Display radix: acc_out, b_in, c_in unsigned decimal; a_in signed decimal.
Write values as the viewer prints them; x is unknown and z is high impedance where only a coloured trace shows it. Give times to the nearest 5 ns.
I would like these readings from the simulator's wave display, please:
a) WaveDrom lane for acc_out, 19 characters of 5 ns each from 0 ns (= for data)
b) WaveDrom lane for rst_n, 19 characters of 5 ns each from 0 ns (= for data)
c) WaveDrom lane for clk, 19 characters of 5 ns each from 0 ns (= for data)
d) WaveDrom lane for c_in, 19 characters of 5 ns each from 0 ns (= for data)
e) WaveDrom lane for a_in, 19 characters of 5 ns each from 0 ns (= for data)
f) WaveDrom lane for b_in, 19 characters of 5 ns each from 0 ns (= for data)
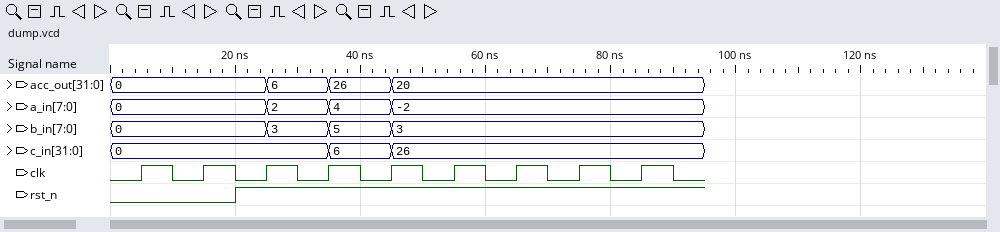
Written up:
{name: 'acc_out', wave: '=....=.=.=.........', data: '0 6 26 20'}
{name: 'rst_n', wave: '0...1..............'}
{name: 'clk', wave: '0101010101010101010'}
{name: 'c_in', wave: '=......=.=.........', data: '0 6 26'}
{name: 'a_in', wave: '=....=.=.=.........', data: '0 2 4 -2'}
{name: 'b_in', wave: '=....=.=.=.........', data: '0 3 5 3'}
